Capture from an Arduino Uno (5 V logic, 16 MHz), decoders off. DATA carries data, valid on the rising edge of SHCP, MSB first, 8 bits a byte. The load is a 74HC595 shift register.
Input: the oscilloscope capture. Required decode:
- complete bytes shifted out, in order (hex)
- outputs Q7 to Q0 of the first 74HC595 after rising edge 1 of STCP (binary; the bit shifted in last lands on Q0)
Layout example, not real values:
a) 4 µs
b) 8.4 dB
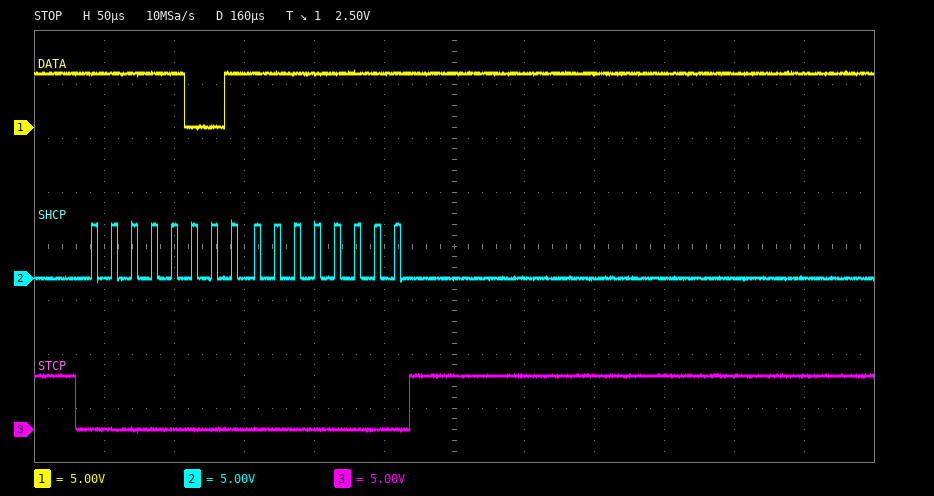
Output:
a) F9 FF
b) 11111111
